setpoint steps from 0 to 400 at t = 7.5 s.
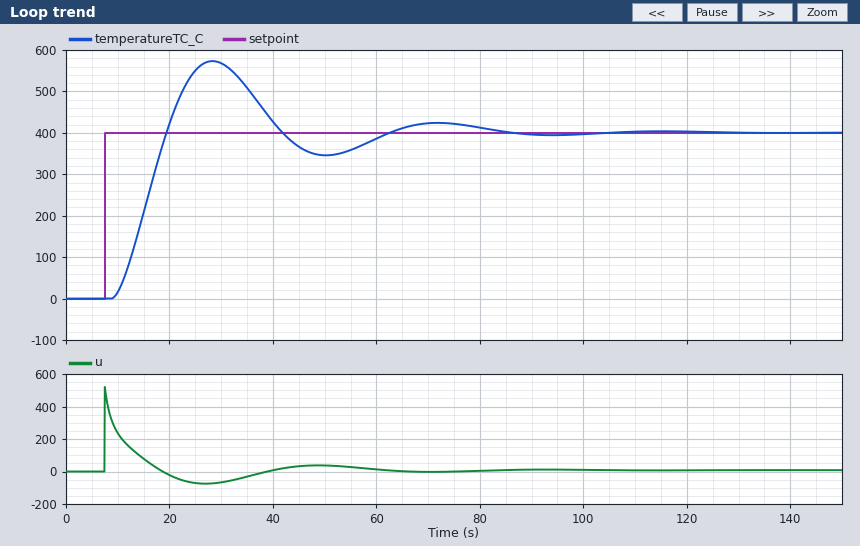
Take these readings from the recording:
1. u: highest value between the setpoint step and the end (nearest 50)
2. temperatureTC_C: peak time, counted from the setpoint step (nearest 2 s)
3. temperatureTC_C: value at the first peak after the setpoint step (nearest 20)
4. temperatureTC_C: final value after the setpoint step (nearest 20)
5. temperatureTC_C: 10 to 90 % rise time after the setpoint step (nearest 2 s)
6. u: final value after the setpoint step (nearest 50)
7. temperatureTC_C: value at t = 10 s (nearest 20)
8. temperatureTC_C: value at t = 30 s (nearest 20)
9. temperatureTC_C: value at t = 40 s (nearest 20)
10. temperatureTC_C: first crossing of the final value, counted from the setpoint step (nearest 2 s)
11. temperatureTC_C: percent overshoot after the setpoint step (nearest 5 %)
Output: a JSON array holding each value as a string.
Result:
["500", "20 s", "580", "400", "8 s", "0", "20", "560", "420", "12 s", "45 %"]
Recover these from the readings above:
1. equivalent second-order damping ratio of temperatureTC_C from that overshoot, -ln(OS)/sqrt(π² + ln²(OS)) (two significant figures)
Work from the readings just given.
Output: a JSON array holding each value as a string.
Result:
["0.25"]
